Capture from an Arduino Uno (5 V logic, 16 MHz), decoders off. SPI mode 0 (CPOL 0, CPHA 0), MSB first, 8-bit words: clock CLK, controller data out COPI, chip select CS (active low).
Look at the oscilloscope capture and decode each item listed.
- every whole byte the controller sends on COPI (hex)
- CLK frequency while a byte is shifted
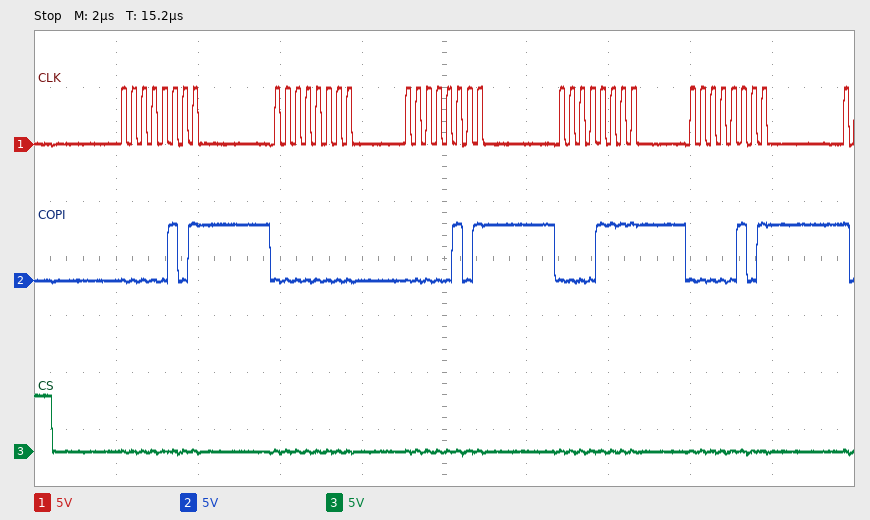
0x05 0x00 0x05 0x0F 0x05
4 MHz
